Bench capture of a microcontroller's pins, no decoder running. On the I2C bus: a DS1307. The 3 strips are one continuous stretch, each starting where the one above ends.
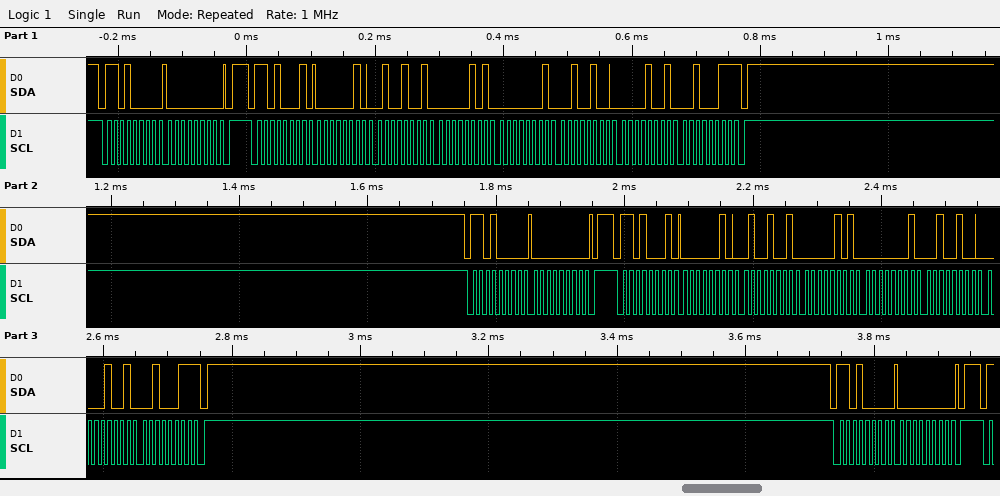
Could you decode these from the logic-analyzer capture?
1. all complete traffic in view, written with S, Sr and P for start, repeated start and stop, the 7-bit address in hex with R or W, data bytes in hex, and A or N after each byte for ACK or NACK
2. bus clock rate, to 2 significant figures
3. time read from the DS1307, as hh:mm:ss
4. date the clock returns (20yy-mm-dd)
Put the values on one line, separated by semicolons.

S 68W A 00 A P S 68R A 02 A 49 A 05 A 01 A 24 A 09 A 23 N P S 68W A 00 A P S 68R A 02 A 49 A 05 A 01 A 24 A 09 A 23 N P S 68W A 00 A P; 100 kHz; 05:49:02; 2023-09-24
